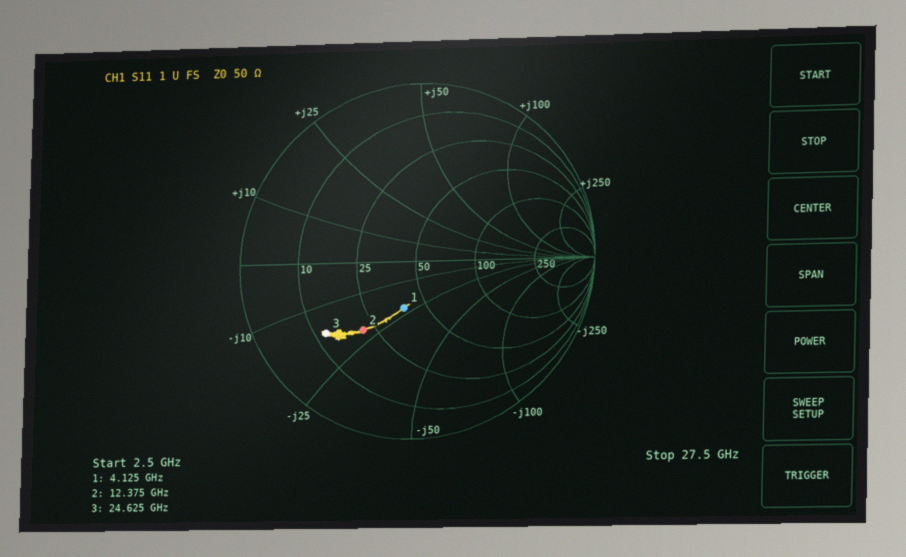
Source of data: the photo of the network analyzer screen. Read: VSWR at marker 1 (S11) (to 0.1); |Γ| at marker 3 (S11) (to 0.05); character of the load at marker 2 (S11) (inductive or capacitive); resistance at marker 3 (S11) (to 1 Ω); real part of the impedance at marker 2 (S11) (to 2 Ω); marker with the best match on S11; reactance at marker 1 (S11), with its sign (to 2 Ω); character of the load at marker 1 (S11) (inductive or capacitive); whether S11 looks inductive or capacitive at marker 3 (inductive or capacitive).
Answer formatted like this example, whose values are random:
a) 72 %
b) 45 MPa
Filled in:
a) 1.7
b) 0.65
c) capacitive
d) 12 Ω
e) 22 Ω
f) marker 1
g) -22 Ω
h) capacitive
i) capacitive
